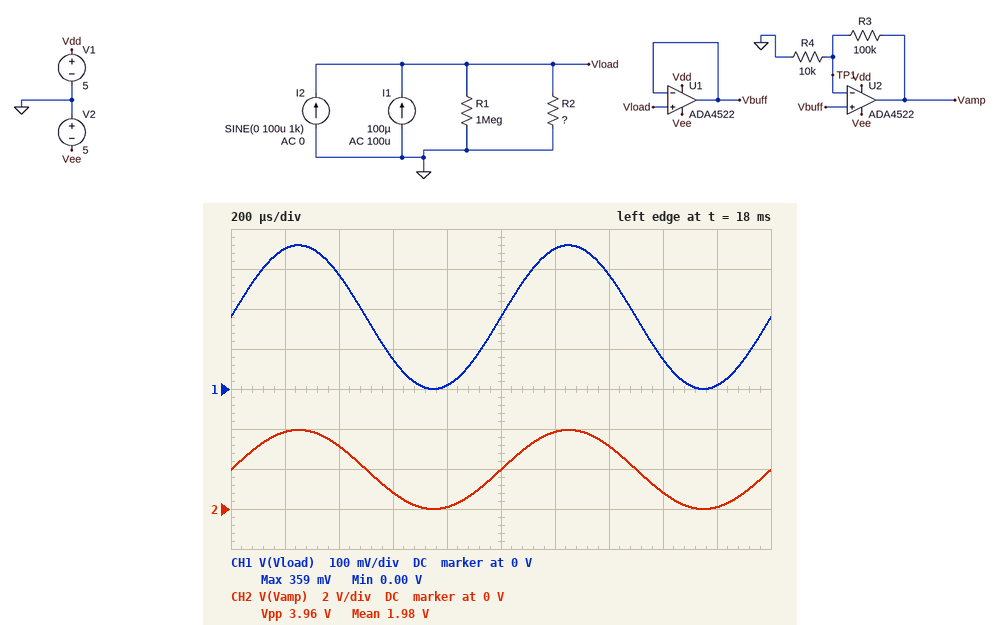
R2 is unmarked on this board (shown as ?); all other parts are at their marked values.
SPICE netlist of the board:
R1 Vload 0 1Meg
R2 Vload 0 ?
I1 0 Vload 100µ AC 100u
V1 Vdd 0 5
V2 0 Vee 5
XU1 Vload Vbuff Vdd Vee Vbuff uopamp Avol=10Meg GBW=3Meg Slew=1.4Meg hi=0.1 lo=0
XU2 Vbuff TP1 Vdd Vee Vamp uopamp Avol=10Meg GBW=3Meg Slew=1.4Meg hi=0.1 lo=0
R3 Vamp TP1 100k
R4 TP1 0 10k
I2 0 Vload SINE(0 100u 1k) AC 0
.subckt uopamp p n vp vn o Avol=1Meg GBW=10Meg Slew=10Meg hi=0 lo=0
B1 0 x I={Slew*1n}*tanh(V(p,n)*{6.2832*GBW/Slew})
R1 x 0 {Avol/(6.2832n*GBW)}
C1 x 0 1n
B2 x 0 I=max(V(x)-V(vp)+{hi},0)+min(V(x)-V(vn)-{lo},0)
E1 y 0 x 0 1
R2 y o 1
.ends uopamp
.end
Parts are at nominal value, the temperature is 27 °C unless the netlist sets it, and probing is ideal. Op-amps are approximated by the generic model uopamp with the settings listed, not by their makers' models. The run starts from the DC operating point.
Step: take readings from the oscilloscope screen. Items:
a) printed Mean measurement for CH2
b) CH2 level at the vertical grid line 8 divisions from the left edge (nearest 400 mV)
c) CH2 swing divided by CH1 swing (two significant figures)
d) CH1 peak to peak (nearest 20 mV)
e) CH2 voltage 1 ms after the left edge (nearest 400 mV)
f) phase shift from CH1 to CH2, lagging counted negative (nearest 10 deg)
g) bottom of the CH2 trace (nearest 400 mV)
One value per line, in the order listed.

1.98 V
800 mV
11
360 mV
2.0 V
0 deg
0 V
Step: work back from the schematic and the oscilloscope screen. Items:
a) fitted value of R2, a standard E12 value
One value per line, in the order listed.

1.8 kΩ
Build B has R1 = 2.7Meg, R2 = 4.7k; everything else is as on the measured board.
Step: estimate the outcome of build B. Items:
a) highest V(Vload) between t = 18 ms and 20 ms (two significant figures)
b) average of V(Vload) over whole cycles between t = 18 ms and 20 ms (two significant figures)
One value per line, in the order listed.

940 mV
470 mV
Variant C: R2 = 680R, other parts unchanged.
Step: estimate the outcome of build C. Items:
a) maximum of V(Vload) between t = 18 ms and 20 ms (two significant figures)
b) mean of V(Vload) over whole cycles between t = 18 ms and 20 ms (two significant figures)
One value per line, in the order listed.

140 mV
68 mV
